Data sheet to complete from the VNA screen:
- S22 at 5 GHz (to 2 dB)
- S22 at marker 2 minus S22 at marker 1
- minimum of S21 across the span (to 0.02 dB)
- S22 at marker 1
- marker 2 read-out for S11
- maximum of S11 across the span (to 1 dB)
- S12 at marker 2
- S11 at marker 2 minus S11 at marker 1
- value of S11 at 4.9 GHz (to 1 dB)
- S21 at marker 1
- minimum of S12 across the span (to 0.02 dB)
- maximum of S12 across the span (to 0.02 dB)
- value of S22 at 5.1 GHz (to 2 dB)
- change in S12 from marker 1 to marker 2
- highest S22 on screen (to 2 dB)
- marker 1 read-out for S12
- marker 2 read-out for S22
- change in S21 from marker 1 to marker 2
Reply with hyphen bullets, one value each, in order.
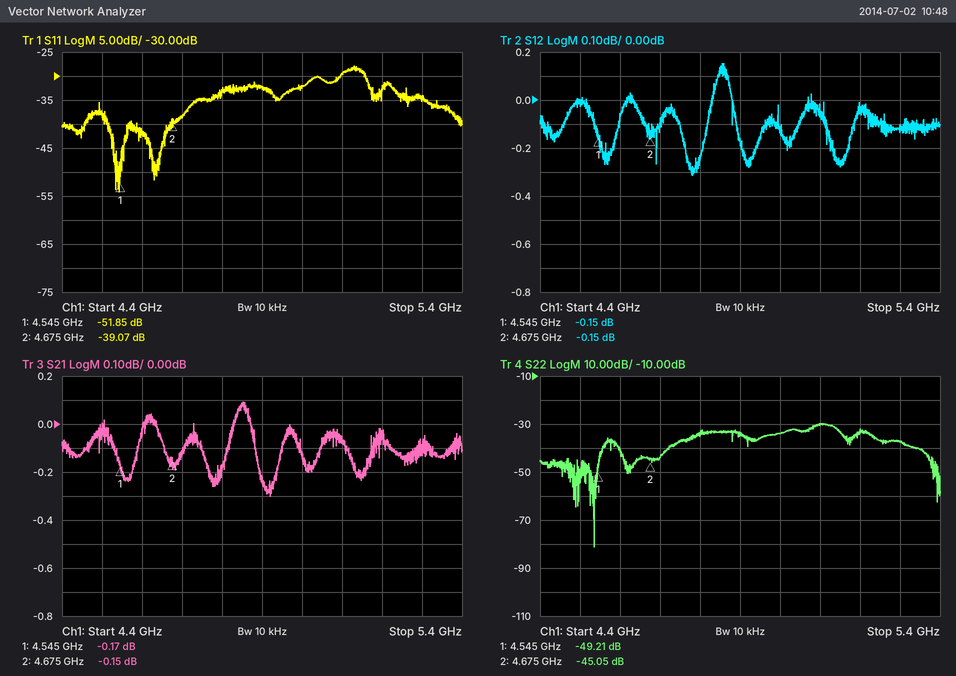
- -34 dB
- 4.16 dB
- -0.30 dB
- -49.21 dB
- -39.07 dB
- -28 dB
- -0.15 dB
- 12.78 dB
- -32 dB
- -0.17 dB
- -0.32 dB
- 0.16 dB
- -30 dB
- 0.00 dB
- -30 dB
- -0.15 dB
- -45.05 dB
- 0.02 dB
